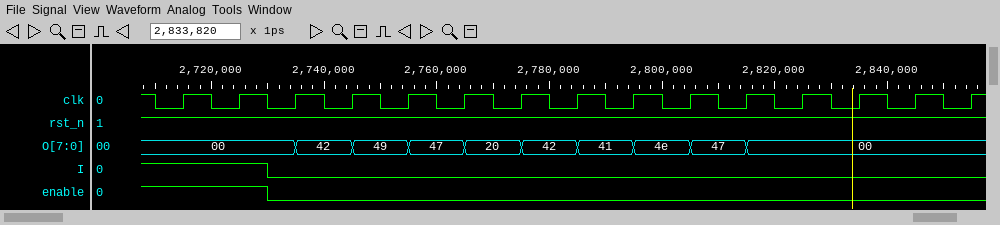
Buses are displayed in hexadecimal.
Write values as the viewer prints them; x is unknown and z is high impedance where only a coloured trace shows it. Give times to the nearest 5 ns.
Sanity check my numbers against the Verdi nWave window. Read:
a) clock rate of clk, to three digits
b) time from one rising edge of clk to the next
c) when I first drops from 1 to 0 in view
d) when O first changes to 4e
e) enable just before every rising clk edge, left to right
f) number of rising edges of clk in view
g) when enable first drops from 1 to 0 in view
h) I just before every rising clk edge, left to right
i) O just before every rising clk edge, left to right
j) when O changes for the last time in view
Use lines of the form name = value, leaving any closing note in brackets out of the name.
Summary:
clock rate of clk, to three digits = 100 MHz
time from one rising edge of clk to the next = 10 ns
when I first drops from 1 to 0 in view = 2730 ns
when O first changes to 4e = 2795 ns
enable just before every rising clk edge, left to right = 1 1 0 0 0 0 0 0 0 0 0 0 0 0 0
number of rising edges of clk in view = 15
when enable first drops from 1 to 0 in view = 2730 ns
I just before every rising clk edge, left to right = 1 1 0 0 0 0 0 0 0 0 0 0 0 0 0
O just before every rising clk edge, left to right = 00, 00, 00, 42, 49, 47, 20, 42, 41, 4e, 47, 00, 00, 00, 00
when O changes for the last time in view = 2815 ns
